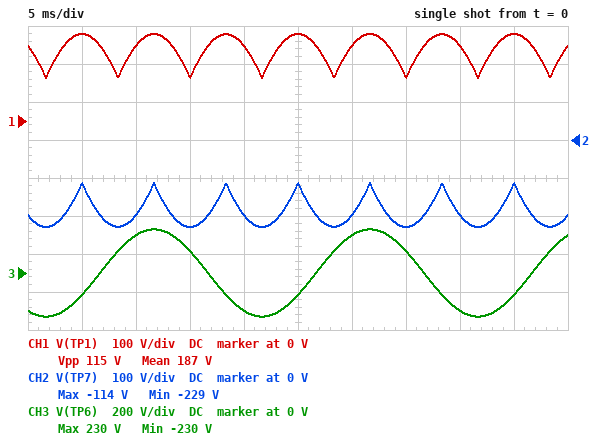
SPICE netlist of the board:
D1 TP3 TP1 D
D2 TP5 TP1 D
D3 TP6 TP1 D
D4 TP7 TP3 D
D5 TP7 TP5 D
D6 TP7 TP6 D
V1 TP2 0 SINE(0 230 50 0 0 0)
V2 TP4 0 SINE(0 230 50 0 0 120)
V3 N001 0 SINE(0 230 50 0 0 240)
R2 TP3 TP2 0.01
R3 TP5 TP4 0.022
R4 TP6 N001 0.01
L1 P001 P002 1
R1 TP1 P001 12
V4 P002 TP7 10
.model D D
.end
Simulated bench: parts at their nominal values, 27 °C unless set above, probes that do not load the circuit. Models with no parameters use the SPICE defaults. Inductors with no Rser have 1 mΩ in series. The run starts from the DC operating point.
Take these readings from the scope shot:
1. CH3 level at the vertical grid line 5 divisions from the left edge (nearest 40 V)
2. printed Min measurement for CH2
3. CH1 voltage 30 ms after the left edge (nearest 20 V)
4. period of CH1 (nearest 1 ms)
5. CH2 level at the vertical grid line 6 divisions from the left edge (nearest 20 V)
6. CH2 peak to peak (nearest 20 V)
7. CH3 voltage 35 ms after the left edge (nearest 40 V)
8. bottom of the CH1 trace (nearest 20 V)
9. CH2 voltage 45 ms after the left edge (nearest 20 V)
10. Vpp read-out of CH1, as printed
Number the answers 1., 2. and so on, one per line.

1. -120 V
2. -229 V
3. 200 V
4. 7 ms
5. -200 V
6. 120 V
7. 120 V
8. 120 V
9. -120 V
10. 115 V
